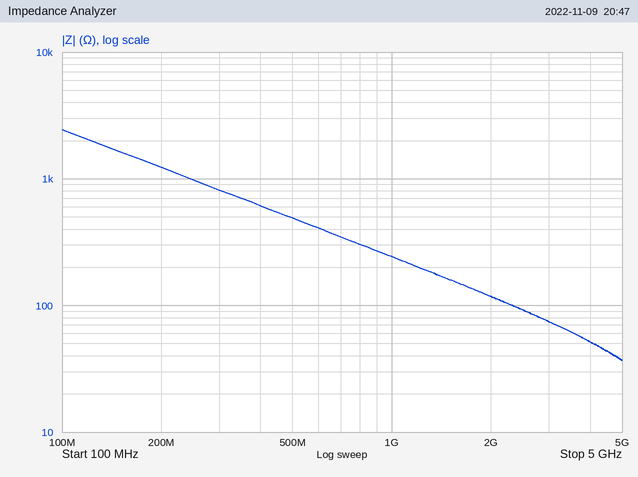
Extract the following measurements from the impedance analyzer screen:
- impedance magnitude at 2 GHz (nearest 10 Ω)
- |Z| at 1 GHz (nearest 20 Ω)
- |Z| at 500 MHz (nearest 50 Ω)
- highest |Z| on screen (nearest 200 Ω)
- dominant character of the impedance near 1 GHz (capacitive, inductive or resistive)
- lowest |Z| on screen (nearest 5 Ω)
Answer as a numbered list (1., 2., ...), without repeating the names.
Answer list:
1. 120 Ω
2. 240 Ω
3. 500 Ω
4. 2.4 kΩ
5. capacitive
6. 35 Ω
